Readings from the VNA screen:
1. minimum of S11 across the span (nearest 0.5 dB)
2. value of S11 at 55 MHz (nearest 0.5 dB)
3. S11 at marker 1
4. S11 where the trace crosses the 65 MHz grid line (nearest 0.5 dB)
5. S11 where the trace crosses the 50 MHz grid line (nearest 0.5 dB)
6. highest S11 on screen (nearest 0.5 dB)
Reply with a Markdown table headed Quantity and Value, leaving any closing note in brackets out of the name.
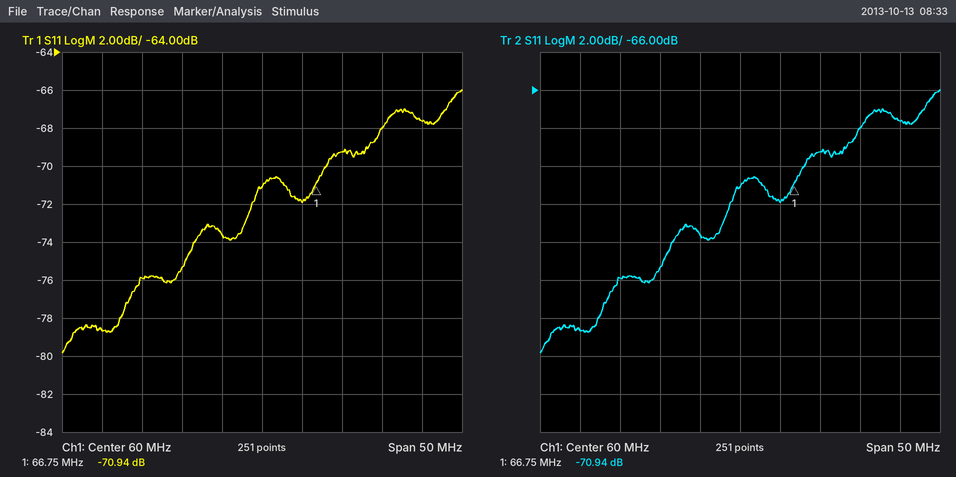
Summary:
| Quantity | Value |
|---|---|
| minimum of S11 across the span | -80.0 dB |
| value of S11 at 55 MHz | -73.5 dB |
| S11 at marker 1 | -70.94 dB |
| S11 where the trace crosses the 65 MHz grid line | -72.0 dB |
| S11 where the trace crosses the 50 MHz grid line | -75.5 dB |
| highest S11 on screen | -66.0 dB |
